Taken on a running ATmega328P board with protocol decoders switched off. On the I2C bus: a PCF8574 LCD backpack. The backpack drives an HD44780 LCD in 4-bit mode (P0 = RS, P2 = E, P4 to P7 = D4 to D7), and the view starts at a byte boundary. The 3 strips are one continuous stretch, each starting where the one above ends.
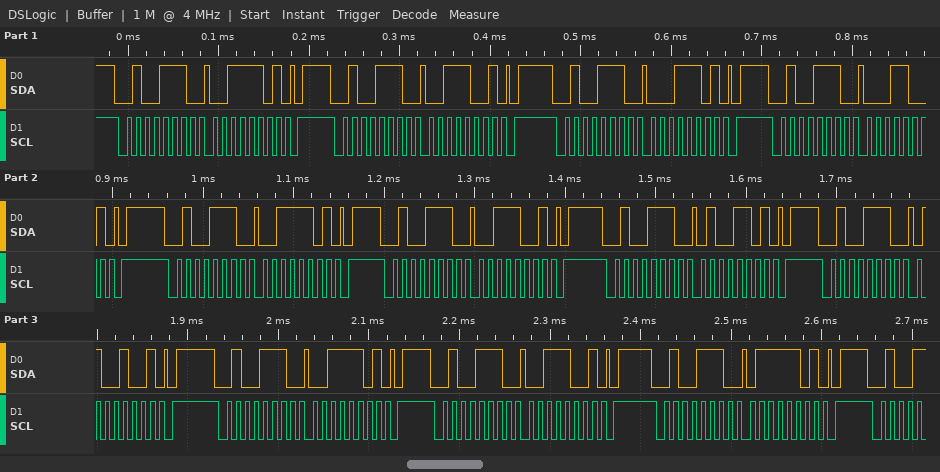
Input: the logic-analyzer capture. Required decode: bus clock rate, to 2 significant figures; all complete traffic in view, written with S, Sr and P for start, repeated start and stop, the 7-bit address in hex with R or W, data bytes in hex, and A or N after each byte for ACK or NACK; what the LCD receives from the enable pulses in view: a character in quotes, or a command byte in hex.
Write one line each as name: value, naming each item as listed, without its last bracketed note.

bus clock rate, to 2 significant figures: 100 kHz
all complete traffic in view, written with S, Sr and P for start, repeated start and stop, the 7-bit address in hex with R or W, data bytes in hex, and A or N after each byte for ACK or NACK: S 27W A 3D A P S 27W A 39 A P S 27W A 1D A P S 27W A 19 A P S 27W A 3D A P S 27W A 39 A P S 27W A 4D A P S 27W A 49 A P S 27W A 3D A P S 27W A 39 A P S 27W A 7D A P
what the LCD receives from the enable pulses in view: a character in quotes, or a command byte in hex: '1' '4'
